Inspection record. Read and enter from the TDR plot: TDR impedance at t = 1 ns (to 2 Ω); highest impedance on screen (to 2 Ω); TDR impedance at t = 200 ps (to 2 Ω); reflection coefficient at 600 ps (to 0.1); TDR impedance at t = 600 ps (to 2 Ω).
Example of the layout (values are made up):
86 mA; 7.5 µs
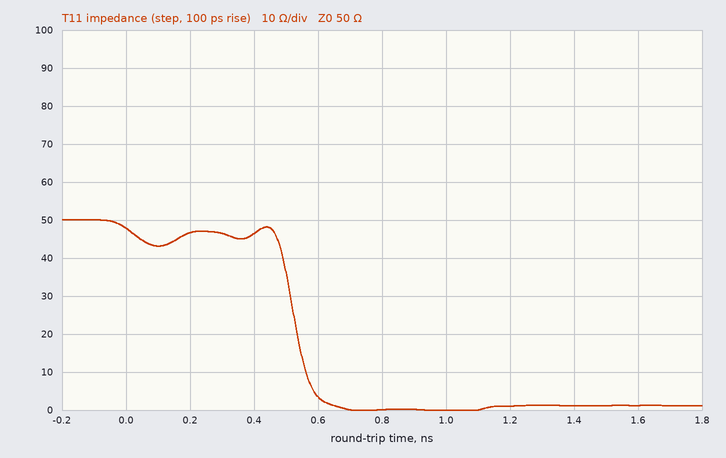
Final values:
0 Ω; 50 Ω; 46 Ω; -0.9; 4 Ω
